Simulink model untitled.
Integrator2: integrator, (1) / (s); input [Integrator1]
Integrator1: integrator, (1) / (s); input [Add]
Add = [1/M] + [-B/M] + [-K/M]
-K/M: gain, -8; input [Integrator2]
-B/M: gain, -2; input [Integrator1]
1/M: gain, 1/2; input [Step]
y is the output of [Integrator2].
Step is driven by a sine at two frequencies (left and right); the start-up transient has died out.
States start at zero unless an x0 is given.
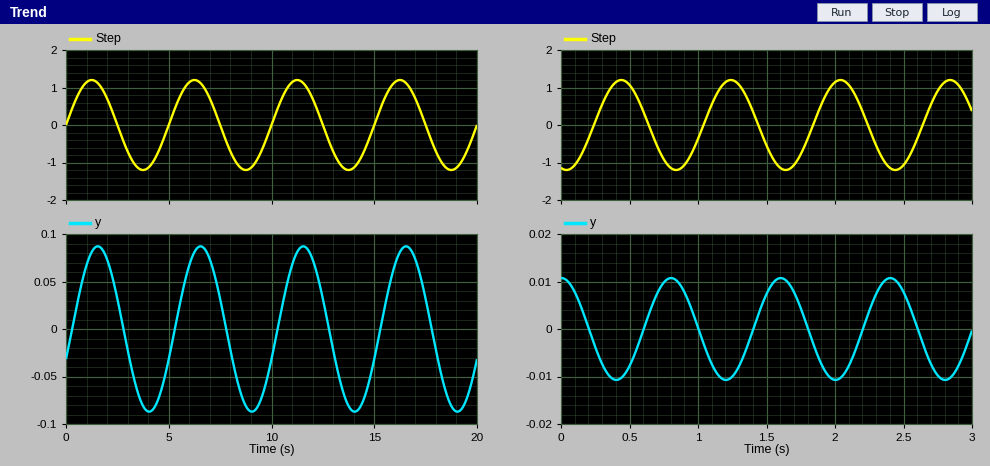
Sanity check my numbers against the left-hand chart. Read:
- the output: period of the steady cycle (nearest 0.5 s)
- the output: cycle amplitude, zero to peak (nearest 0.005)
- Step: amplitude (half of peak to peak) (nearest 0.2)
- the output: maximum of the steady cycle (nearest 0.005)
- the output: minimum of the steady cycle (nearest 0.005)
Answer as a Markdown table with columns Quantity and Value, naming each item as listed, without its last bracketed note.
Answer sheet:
| Quantity | Value |
|---|---|
| the output: period of the steady cycle | 5.0 s |
| the output: cycle amplitude, zero to peak | 0.085 |
| Step: amplitude (half of peak to peak) | 1.2 |
| the output: maximum of the steady cycle | 0.085 |
| the output: minimum of the steady cycle | -0.085 |
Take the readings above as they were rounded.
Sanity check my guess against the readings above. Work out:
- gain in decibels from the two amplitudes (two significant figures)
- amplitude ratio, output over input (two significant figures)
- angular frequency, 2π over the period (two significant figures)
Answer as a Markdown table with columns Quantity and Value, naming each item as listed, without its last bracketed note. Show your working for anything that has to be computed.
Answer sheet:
| Quantity | Value |
|---|---|
| gain in decibels from the two amplitudes | 20 log10(0.085 / 1.2) = -23 dB |
| amplitude ratio, output over input | 0.085 / 1.2 = 0.071 |
| angular frequency, 2π over the period | 2π / 5 = 1.3 rad/s |
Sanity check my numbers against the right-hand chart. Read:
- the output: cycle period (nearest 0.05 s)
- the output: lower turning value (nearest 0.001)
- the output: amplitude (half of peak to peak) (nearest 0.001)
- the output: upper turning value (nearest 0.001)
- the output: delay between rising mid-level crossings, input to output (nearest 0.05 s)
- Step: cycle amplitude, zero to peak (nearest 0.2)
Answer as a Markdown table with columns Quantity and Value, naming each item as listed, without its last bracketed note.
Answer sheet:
| Quantity | Value |
|---|---|
| the output: cycle period | 0.80 s |
| the output: lower turning value | -0.011 |
| the output: amplitude (half of peak to peak) | 0.011 |
| the output: upper turning value | 0.011 |
| the output: delay between rising mid-level crossings, input to output | 0.35 s |
| Step: cycle amplitude, zero to peak | 1.2 |
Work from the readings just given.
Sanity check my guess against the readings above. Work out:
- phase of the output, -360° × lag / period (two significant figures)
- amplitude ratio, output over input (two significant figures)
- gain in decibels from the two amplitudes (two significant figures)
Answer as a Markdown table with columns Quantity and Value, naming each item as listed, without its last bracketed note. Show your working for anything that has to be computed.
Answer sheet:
| Quantity | Value |
|---|---|
| phase of the output, -360° × lag / period | -360 × 0.35 / 0.8 = -160° |
| amplitude ratio, output over input | 0.011 / 1.2 = 0.0092 |
| gain in decibels from the two amplitudes | 20 log10(0.011 / 1.2) = -41 dB |
